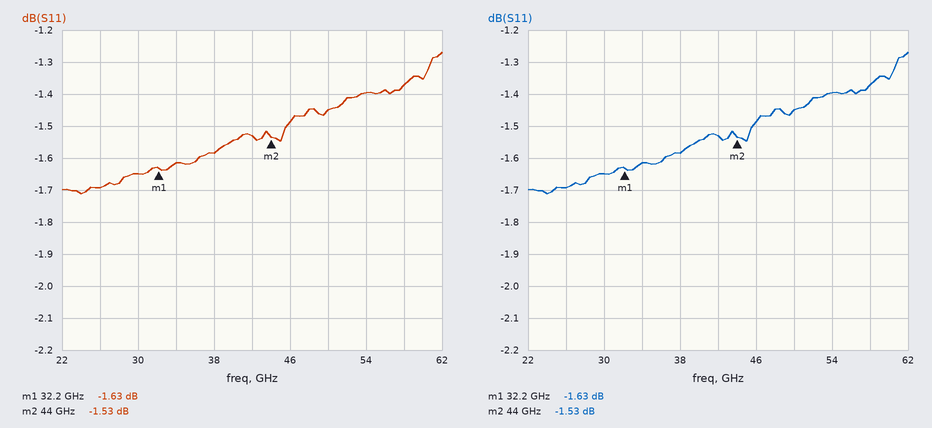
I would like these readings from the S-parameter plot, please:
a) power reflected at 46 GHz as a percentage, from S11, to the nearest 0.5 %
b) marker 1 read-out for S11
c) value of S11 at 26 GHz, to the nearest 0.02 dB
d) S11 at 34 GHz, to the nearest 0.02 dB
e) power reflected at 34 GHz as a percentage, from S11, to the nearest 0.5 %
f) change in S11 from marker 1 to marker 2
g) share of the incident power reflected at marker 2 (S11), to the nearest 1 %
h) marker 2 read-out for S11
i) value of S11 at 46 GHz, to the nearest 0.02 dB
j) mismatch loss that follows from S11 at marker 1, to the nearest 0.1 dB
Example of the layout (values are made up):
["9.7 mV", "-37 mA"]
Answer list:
["71.0 %", "-1.63 dB", "-1.70 dB", "-1.62 dB", "69.0 %", "0.10 dB", "70 %", "-1.53 dB", "-1.48 dB", "5.0 dB"]
